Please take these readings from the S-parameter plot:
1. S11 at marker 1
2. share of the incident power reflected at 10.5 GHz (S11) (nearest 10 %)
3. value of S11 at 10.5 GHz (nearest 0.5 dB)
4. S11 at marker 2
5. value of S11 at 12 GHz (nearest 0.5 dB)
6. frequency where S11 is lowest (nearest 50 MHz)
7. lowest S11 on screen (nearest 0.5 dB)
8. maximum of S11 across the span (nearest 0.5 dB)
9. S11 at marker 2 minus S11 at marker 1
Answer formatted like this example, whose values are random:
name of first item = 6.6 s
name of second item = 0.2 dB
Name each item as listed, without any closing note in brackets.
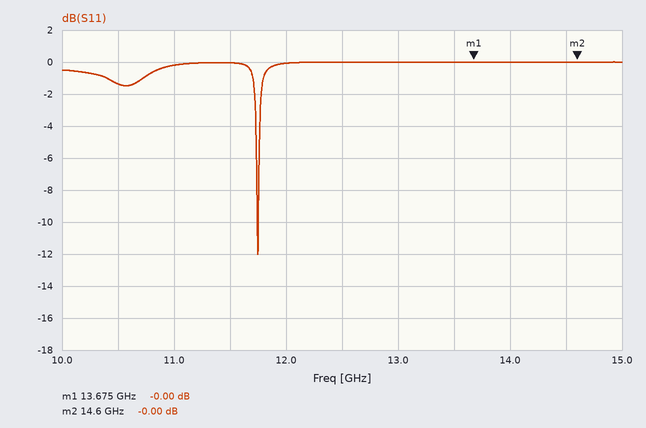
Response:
S11 at marker 1 = -0.00 dB
share of the incident power reflected at 10.5 GHz (S11) = 70 %
value of S11 at 10.5 GHz = -1.5 dB
S11 at marker 2 = -0.00 dB
value of S11 at 12 GHz = 0.0 dB
frequency where S11 is lowest = 11.75 GHz
lowest S11 on screen = -12.0 dB
maximum of S11 across the span = 0.0 dB
S11 at marker 2 minus S11 at marker 1 = 0.00 dB
